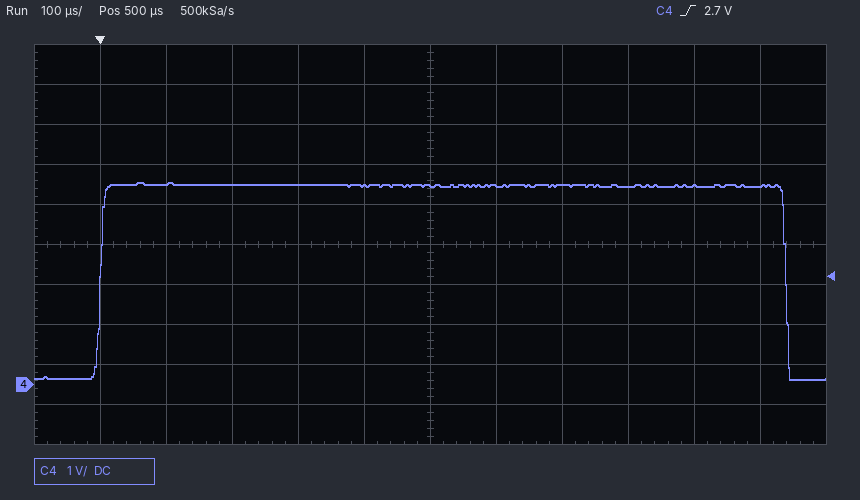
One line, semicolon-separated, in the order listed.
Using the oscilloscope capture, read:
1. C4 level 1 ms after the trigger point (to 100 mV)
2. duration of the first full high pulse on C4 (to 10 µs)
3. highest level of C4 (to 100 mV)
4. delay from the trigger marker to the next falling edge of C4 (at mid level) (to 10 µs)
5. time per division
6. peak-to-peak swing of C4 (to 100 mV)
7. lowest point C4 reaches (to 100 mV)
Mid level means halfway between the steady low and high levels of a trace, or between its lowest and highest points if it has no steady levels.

5.0 V; 1.04 ms; 5.0 V; 1.04 ms; 100 µs; 4.9 V; 100 mV
